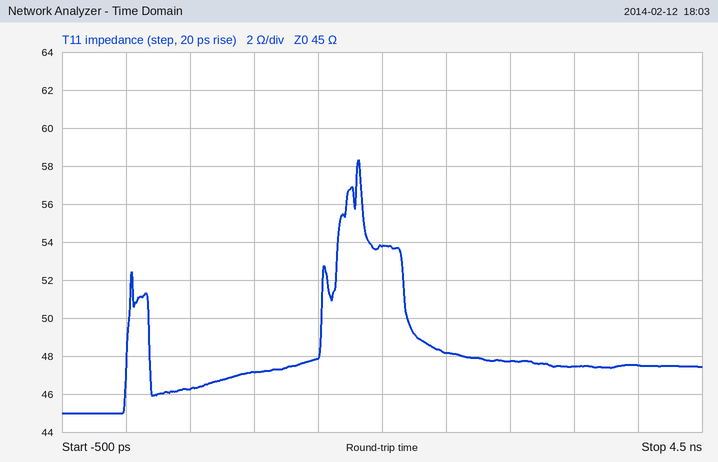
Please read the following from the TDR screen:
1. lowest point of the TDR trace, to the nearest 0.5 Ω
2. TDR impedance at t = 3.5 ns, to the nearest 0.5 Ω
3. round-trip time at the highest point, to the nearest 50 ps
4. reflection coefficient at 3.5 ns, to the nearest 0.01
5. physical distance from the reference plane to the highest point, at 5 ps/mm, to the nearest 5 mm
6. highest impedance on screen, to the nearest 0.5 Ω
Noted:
45.0 Ω
47.5 Ω
1.80 ns
+0.03
180 mm
58.5 Ω
